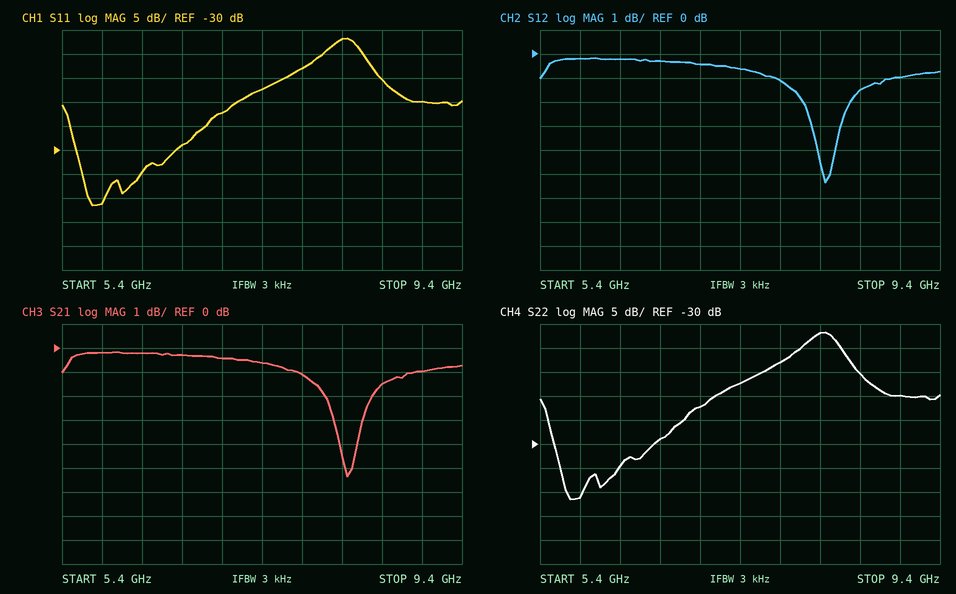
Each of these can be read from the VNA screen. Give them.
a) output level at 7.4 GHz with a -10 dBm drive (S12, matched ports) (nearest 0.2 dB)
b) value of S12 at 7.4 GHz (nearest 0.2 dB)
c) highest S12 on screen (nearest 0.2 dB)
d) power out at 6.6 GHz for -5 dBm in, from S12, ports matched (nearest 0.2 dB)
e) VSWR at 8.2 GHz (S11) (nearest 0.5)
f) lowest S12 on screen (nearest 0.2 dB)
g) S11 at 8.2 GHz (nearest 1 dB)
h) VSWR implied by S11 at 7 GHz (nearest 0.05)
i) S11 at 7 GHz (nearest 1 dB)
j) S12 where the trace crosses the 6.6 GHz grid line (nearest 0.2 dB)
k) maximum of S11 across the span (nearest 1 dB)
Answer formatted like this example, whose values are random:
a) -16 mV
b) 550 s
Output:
a) -10.6 dBm
b) -0.6 dB
c) -0.2 dB
d) -5.2 dBm
e) 2.5
f) -5.4 dB
g) -7 dB
h) 1.15
i) -22 dB
j) -0.2 dB
k) -7 dB
